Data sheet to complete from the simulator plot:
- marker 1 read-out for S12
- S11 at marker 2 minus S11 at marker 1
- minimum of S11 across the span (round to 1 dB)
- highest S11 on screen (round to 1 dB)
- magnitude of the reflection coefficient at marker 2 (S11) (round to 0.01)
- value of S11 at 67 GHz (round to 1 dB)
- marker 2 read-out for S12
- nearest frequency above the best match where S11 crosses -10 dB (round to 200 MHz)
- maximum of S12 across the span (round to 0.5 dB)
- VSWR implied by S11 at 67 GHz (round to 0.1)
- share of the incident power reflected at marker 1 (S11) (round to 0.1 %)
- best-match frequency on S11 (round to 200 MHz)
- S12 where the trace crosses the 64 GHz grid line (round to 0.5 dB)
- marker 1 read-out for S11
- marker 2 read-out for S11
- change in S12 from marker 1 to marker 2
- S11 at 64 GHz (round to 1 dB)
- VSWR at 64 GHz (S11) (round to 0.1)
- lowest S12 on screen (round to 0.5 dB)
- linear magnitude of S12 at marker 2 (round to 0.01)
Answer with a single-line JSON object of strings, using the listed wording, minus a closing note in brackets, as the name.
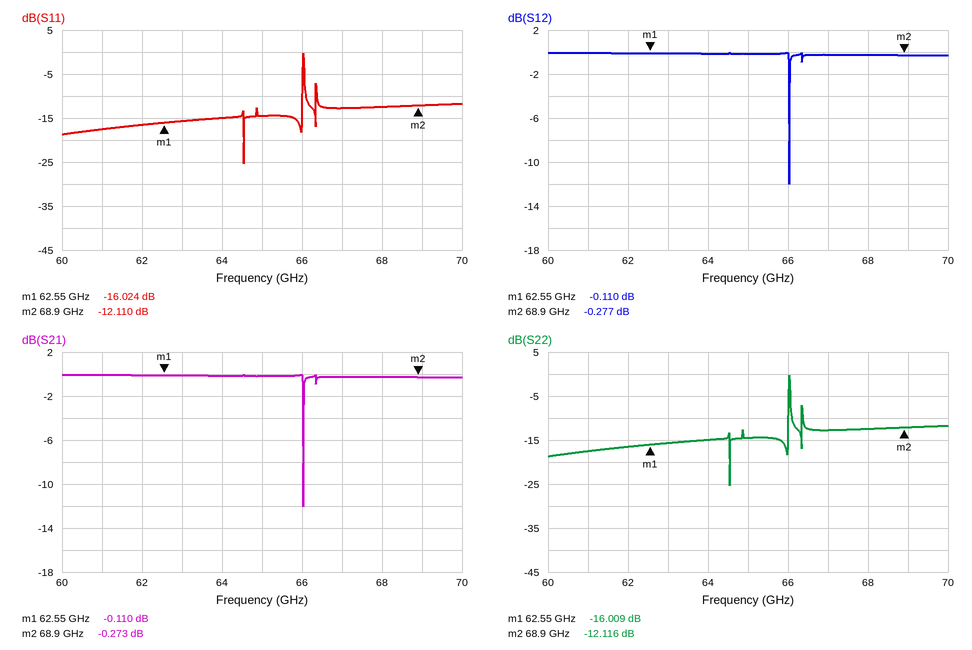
{"marker 1 read-out for S12": "-0.110 dB", "S11 at marker 2 minus S11 at marker 1": "3.914 dB", "minimum of S11 across the span": "-25 dB", "highest S11 on screen": "0 dB", "magnitude of the reflection coefficient at marker 2 (S11)": "0.25", "value of S11 at 67 GHz": "-13 dB", "marker 2 read-out for S12": "-0.277 dB", "nearest frequency above the best match where S11 crosses -10 dB": "66.0 GHz", "maximum of S12 across the span": "0.0 dB", "VSWR implied by S11 at 67 GHz": "1.6", "share of the incident power reflected at marker 1 (S11)": "2.5 %", "best-match frequency on S11": "64.6 GHz", "S12 where the trace crosses the 64 GHz grid line": "0.0 dB", "marker 1 read-out for S11": "-16.024 dB", "marker 2 read-out for S11": "-12.110 dB", "change in S12 from marker 1 to marker 2": "-0.167 dB", "S11 at 64 GHz": "-15 dB", "VSWR at 64 GHz (S11)": "1.4", "lowest S12 on screen": "-12.0 dB", "linear magnitude of S12 at marker 2": "0.97"}
